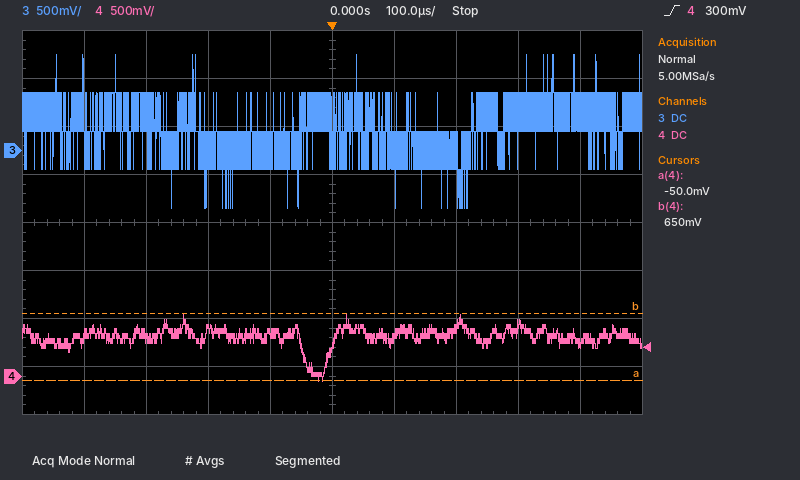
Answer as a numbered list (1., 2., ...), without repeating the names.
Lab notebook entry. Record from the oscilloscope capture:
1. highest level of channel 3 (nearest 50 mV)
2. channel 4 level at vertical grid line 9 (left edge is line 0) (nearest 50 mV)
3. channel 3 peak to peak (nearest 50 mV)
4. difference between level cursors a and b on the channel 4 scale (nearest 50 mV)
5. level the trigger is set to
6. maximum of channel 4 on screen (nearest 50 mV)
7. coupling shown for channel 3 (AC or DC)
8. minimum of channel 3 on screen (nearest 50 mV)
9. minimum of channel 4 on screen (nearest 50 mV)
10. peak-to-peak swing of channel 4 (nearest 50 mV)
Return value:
1. 1.00 V
2. 350 mV
3. 1.60 V
4. 700 mV
5. 300 mV
6. 650 mV
7. DC
8. -600 mV
9. -50 mV
10. 700 mV
